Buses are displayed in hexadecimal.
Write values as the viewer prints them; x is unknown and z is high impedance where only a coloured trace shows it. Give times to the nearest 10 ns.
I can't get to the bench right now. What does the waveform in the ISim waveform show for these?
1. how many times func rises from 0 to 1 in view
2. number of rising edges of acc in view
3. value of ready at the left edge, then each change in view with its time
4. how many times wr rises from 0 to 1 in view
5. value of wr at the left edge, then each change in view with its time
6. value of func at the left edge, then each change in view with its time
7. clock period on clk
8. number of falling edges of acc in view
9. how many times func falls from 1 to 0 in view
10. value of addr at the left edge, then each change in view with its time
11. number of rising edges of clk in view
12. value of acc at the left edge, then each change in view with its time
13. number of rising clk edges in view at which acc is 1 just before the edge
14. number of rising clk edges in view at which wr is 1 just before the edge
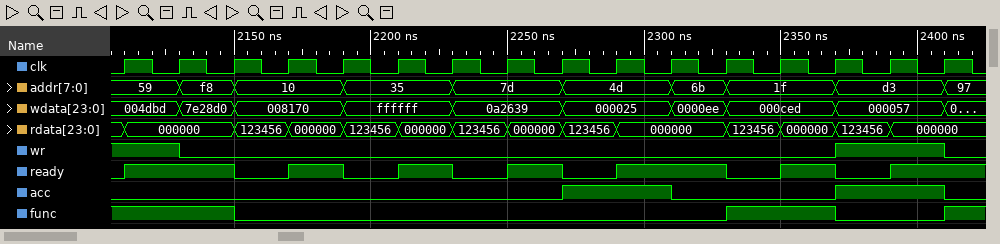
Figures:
2
2
0, 1 at 2110 ns, 0 at 2150 ns, 1 at 2170 ns, 0 at 2190 ns, 1 at 2210 ns, 0 at 2230 ns, 1 at 2250 ns, 0 at 2270 ns, 1 at 2290 ns, 0 at 2330 ns, 1 at 2350 ns, 0 at 2370 ns, 1 at 2390 ns
1
1, 0 at 2130 ns, 1 at 2370 ns, 0 at 2410 ns
1, 0 at 2150 ns, 1 at 2330 ns, 0 at 2370 ns, 1 at 2410 ns
20 ns
2
2
59, f8 at 2130 ns, 10 at 2150 ns, 35 at 2190 ns, 7d at 2230 ns, 4d at 2270 ns, 6b at 2310 ns, 1f at 2330 ns, d3 at 2370 ns, 97 at 2410 ns
16
0, 1 at 2270 ns, 0 at 2310 ns, 1 at 2370 ns, 0 at 2410 ns
4
4
